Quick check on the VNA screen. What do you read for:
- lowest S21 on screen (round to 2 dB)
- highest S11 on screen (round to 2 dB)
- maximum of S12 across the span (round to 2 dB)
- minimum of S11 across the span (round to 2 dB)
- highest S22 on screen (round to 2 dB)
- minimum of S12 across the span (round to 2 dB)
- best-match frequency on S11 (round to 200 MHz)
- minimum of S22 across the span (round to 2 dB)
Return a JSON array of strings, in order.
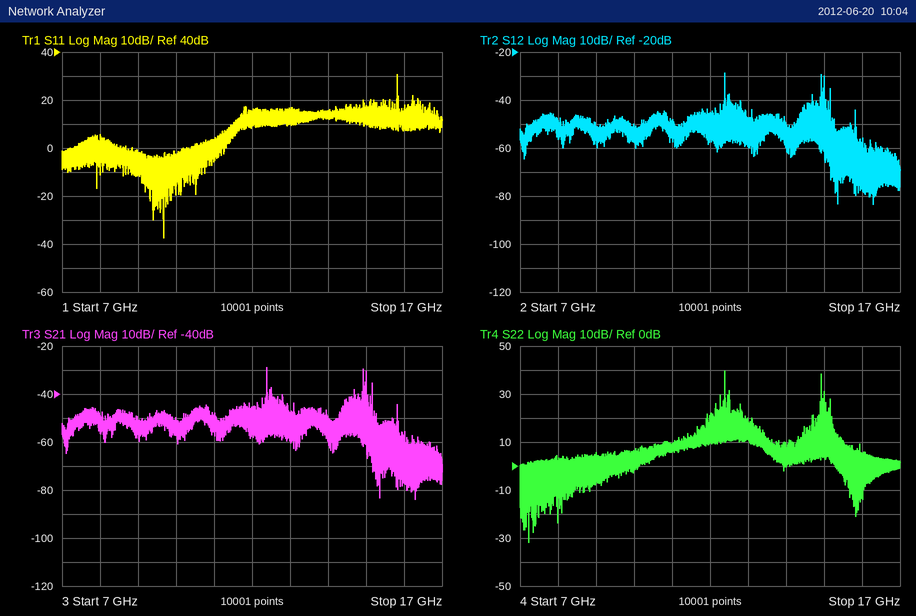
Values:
["-84 dB", "30 dB", "-28 dB", "-38 dB", "40 dB", "-84 dB", "9.6 GHz", "-32 dB"]
